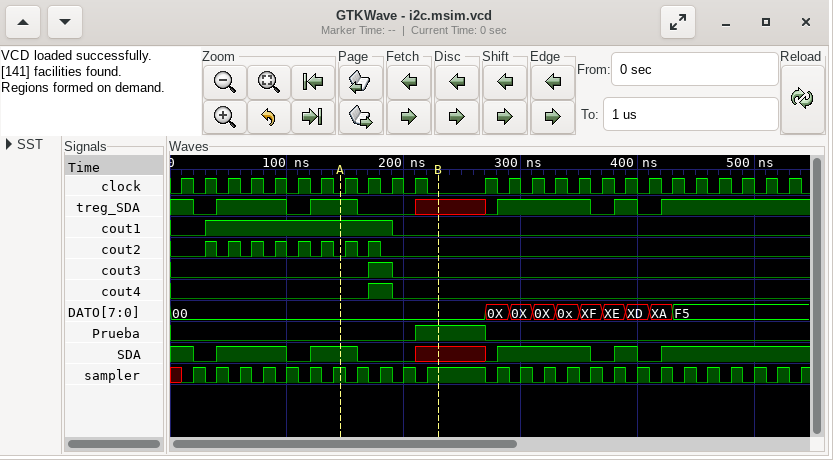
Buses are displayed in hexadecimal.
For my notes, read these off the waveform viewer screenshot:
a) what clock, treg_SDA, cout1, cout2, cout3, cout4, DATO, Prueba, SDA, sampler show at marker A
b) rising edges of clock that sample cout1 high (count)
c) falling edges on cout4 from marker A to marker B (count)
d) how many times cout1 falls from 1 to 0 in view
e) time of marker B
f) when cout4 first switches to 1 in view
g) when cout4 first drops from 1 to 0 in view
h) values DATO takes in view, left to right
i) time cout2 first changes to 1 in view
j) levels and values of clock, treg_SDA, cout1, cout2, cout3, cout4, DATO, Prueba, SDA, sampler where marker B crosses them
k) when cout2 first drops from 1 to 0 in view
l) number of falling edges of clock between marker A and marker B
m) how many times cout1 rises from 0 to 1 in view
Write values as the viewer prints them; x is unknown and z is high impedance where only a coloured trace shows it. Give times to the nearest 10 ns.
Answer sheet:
clock=0, treg_SDA=1, cout1=1, cout2=0, cout3=0, cout4=0, DATO=00, Prueba=0, SDA=1, sampler=1
8
1
1
230 ns
170 ns
190 ns
00, 0X, 0X, 0X, 0x, XF, XE, XD, XA, F5
30 ns
clock=0, treg_SDA=x, cout1=0, cout2=0, cout3=0, cout4=0, DATO=00, Prueba=1, SDA=x, sampler=1
40 ns
4
1
